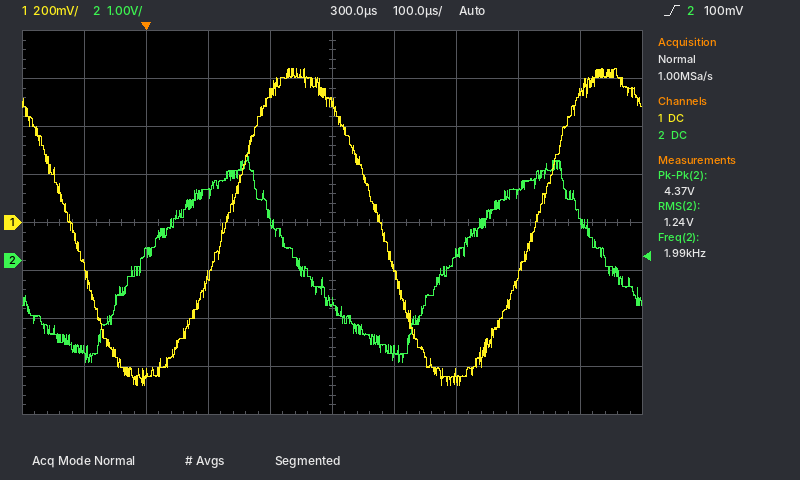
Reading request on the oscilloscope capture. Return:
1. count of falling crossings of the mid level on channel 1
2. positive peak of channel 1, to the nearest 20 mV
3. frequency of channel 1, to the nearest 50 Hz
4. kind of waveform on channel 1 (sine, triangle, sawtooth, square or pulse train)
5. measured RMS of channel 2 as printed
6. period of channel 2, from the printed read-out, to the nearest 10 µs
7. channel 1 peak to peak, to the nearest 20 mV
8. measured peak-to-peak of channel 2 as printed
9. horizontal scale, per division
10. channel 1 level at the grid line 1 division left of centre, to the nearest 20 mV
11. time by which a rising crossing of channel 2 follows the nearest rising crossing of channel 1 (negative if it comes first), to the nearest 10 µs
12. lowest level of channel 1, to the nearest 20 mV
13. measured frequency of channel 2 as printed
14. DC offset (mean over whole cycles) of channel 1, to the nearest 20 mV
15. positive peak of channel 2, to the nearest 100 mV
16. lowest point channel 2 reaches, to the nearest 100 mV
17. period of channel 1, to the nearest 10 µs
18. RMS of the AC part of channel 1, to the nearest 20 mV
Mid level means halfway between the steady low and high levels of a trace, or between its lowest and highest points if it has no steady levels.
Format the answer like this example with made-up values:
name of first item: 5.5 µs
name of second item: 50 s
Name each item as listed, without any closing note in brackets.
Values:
count of falling crossings of the mid level on channel 1: 2
positive peak of channel 1, to the nearest 20 mV: 640 mV
frequency of channel 1, to the nearest 50 Hz: 2.00 kHz
kind of waveform on channel 1: sine
measured RMS of channel 2 as printed: 1.24 V
period of channel 2, from the printed read-out, to the nearest 10 µs: 500 µs
channel 1 peak to peak, to the nearest 20 mV: 1.32 V
measured peak-to-peak of channel 2 as printed: 4.37 V
horizontal scale, per division: 100 µs
channel 1 level at the grid line 1 division left of centre, to the nearest 20 mV: 540 mV
time by which a rising crossing of channel 2 follows the nearest rising crossing of channel 1 (negative if it comes first), to the nearest 10 µs: -130 µs
lowest level of channel 1, to the nearest 20 mV: -680 mV
measured frequency of channel 2 as printed: 1.99 kHz
DC offset (mean over whole cycles) of channel 1, to the nearest 20 mV: -20 mV
positive peak of channel 2, to the nearest 100 mV: 2.3 V
lowest point channel 2 reaches, to the nearest 100 mV: -2.1 V
period of channel 1, to the nearest 10 µs: 500 µs
RMS of the AC part of channel 1, to the nearest 20 mV: 460 mV
